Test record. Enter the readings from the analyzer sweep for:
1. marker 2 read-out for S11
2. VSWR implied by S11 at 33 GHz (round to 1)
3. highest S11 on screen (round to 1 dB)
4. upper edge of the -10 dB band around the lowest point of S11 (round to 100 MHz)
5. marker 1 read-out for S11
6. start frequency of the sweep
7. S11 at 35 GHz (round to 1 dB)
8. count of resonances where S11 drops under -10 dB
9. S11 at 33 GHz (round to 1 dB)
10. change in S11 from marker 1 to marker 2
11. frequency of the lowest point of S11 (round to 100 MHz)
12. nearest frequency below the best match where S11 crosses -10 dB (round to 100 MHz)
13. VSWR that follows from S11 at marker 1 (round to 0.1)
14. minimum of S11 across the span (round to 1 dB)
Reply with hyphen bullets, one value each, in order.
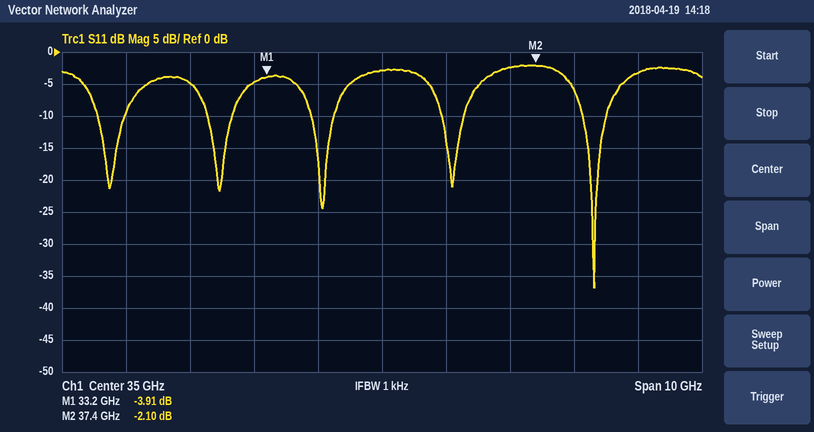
- -2.10 dB
- 4
- -2 dB
- 38.5 GHz
- -3.91 dB
- 30 GHz
- -3 dB
- 5
- -5 dB
- 1.81 dB
- 38.3 GHz
- 38.1 GHz
- 4.5
- -37 dB
